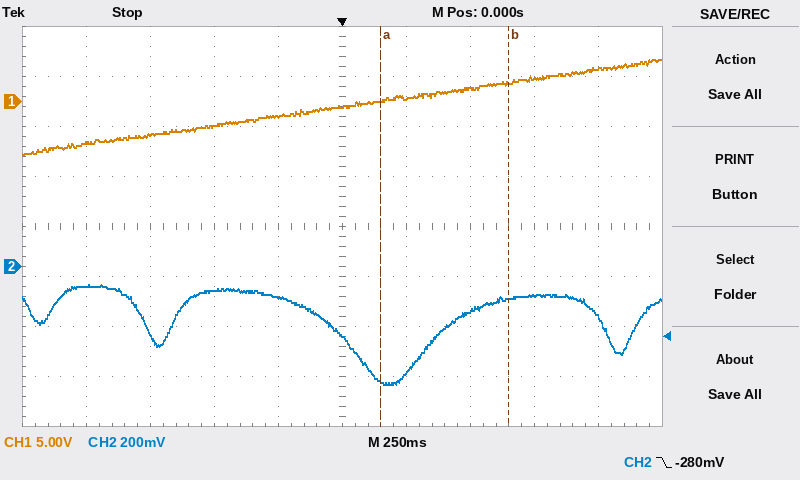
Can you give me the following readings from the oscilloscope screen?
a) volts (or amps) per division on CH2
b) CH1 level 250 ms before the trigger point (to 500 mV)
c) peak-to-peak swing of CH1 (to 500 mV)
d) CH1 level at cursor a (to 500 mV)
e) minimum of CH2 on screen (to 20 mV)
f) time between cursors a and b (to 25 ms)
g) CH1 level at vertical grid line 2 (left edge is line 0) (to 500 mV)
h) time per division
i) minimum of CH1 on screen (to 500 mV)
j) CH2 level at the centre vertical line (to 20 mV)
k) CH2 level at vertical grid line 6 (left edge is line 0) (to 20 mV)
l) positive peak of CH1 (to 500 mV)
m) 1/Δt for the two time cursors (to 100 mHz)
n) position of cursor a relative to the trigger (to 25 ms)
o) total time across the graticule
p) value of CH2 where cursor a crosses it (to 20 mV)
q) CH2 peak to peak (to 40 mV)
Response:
200 mV
-1.5 V
9.5 V
0.0 V
-480 mV
500 ms
-3.5 V
250 ms
-5.5 V
-280 mV
-420 mV
4.0 V
2.0 Hz
+150 ms
2.5 s
-460 mV
400 mV
